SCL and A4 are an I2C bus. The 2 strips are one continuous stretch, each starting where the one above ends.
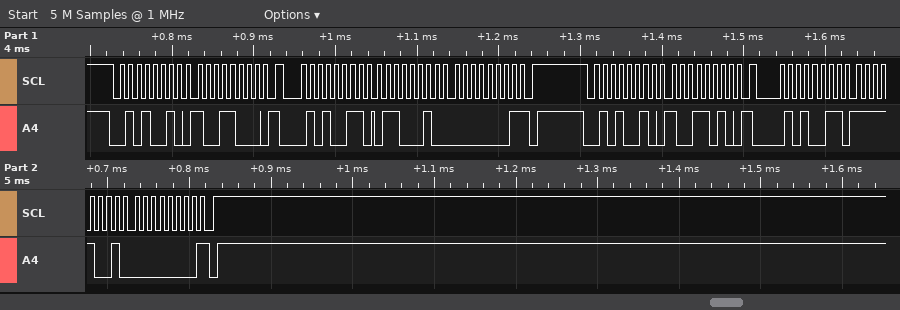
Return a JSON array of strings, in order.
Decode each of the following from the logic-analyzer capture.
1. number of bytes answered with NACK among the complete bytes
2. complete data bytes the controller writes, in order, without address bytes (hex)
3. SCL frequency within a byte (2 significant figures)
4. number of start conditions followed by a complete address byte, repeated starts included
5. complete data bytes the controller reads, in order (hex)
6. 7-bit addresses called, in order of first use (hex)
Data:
["2", "98 9A", "100 kHz", "4", "62 01 F9 00", "0x29"]
